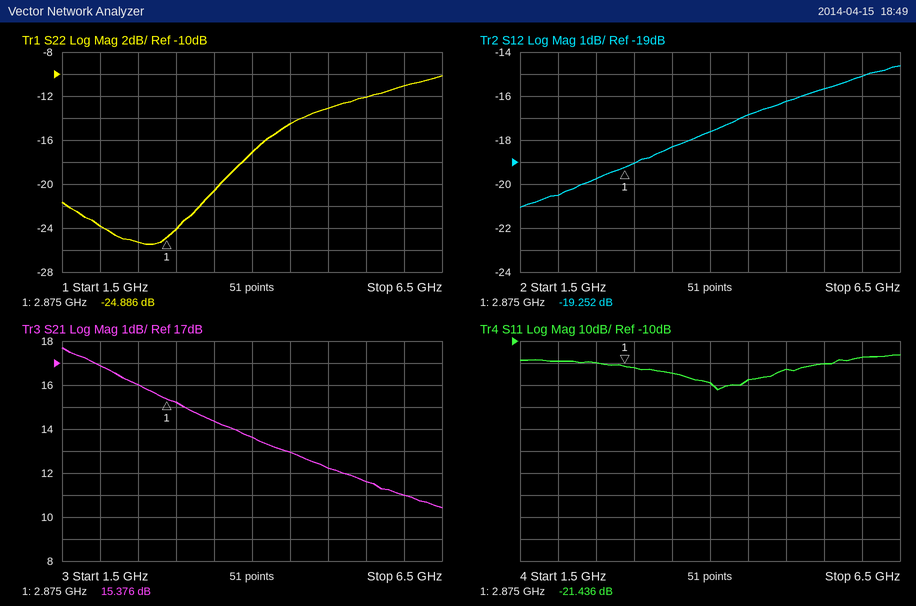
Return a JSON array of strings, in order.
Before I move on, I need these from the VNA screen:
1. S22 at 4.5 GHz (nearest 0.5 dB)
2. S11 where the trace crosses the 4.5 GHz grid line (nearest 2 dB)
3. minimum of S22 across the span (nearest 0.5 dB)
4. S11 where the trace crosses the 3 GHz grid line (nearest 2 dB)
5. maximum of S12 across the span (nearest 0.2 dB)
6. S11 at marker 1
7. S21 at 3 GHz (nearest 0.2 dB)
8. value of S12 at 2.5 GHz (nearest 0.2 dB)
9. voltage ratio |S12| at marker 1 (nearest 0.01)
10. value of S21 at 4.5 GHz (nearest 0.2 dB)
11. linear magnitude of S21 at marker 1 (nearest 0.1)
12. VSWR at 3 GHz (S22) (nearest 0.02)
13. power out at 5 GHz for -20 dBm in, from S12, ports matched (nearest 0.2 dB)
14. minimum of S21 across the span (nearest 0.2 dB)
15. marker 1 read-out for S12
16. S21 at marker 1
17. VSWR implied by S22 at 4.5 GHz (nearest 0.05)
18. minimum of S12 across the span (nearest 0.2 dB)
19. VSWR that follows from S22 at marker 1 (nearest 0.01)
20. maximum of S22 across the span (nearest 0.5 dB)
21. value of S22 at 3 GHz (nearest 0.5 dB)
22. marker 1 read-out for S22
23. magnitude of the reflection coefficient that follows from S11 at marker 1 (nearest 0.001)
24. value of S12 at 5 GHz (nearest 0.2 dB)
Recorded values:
["-14.5 dB", "-28 dB", "-25.5 dB", "-22 dB", "-14.6 dB", "-21.436 dB", "15.2 dB", "-19.8 dB", "0.11", "13.0 dB", "5.9", "1.14", "-36.2 dBm", "10.4 dB", "-19.252 dB", "15.376 dB", "1.45", "-21.0 dB", "1.12", "-10.0 dB", "-24.0 dB", "-24.886 dB", "0.085", "-16.2 dB"]
